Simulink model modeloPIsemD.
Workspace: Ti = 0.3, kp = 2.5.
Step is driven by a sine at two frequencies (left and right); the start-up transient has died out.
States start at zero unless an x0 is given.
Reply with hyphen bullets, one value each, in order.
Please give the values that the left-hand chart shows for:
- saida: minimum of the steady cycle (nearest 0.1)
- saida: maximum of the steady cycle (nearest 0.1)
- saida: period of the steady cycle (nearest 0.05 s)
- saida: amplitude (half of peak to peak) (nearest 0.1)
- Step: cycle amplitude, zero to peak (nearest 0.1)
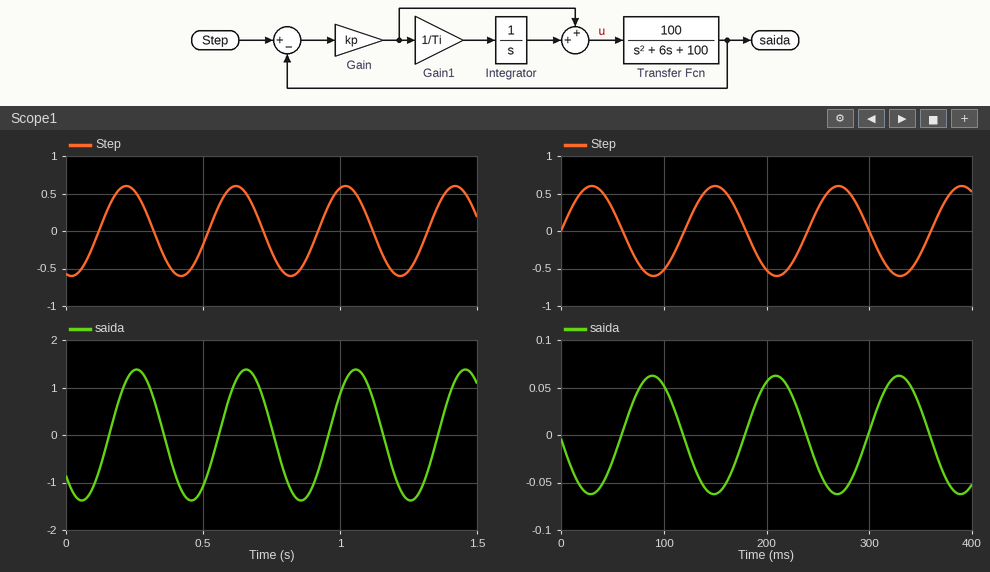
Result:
- -1.4
- 1.4
- 0.40 s
- 1.4
- 0.6
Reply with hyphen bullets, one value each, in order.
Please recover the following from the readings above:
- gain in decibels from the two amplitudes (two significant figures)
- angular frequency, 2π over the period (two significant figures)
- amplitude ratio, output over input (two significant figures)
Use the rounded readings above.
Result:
- 7.4 dB
- 16 rad/s
- 2.3
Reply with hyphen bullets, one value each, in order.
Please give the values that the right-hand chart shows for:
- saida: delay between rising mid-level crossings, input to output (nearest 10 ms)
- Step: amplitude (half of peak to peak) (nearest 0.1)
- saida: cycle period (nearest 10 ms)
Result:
- 60 ms
- 0.6
- 120 ms
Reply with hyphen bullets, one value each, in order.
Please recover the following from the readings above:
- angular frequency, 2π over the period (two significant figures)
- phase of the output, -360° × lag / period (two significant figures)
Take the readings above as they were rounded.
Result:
- 0.052 rad/ms
- -180°
